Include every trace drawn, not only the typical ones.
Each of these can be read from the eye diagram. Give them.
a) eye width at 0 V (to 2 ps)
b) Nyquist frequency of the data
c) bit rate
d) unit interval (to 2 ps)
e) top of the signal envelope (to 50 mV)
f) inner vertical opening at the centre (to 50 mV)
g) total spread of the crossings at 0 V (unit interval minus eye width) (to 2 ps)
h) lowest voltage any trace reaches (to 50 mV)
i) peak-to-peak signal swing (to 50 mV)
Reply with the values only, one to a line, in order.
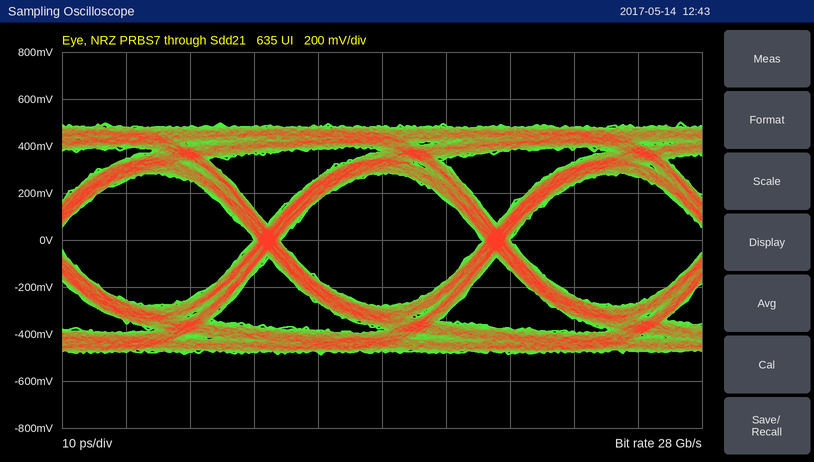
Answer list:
32 ps
14 GHz
28 Gb/s
36 ps
500 mV
550 mV
4 ps
-500 mV
1.00 V
